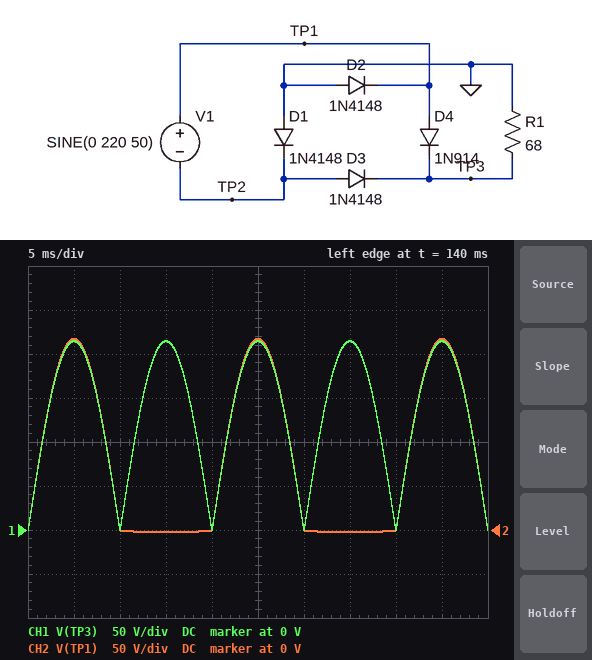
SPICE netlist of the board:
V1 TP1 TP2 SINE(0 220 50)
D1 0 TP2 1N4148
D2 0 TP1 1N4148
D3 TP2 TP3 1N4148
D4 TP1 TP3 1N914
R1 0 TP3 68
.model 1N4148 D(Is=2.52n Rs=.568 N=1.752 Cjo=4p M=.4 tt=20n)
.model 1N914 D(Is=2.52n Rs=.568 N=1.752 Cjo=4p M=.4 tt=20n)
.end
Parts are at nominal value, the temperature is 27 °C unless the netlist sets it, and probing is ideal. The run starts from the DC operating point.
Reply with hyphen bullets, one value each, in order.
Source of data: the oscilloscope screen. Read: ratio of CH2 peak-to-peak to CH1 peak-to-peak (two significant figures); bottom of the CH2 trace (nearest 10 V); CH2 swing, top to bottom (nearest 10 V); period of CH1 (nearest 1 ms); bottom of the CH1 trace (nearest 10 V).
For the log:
- 1.0
- 0 V
- 220 V
- 10 ms
- 0 V
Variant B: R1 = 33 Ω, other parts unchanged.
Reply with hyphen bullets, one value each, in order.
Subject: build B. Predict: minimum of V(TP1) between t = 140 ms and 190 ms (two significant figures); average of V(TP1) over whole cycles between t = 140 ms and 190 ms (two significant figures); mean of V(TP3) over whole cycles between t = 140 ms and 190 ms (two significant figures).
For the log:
- -4.6 V
- 67 V
- 130 V
